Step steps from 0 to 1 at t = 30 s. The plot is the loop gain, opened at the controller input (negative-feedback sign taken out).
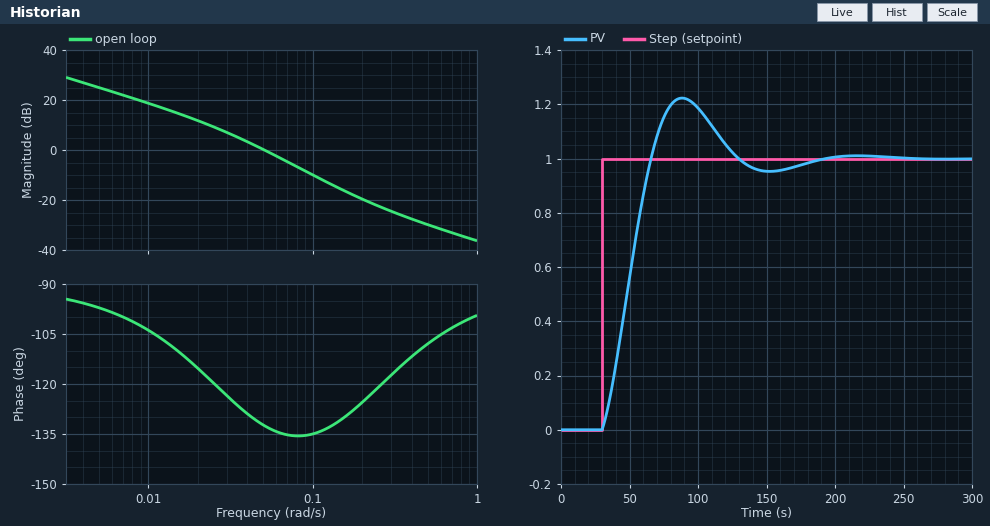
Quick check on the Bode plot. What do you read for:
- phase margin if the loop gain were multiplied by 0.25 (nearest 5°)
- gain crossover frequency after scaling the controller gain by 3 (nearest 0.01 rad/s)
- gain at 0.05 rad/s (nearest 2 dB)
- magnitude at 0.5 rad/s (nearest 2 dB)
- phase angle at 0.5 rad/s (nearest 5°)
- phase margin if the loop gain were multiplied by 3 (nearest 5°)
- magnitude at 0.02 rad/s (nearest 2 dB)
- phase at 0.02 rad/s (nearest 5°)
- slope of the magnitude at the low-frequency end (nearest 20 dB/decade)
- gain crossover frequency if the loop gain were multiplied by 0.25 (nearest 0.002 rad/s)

65°
0.10 rad/s
0 dB
-30 dB
-110°
45°
12 dB
-115°
-20 dB/decade
0.020 rad/s
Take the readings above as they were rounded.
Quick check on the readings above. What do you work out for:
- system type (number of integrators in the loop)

1
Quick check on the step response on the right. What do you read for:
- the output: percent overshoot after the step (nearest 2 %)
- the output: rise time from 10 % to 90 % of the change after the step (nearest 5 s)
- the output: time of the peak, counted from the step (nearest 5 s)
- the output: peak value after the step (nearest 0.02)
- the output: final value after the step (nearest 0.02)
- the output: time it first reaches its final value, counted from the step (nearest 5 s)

22 %
25 s
60 s
1.22
1.00
35 s
